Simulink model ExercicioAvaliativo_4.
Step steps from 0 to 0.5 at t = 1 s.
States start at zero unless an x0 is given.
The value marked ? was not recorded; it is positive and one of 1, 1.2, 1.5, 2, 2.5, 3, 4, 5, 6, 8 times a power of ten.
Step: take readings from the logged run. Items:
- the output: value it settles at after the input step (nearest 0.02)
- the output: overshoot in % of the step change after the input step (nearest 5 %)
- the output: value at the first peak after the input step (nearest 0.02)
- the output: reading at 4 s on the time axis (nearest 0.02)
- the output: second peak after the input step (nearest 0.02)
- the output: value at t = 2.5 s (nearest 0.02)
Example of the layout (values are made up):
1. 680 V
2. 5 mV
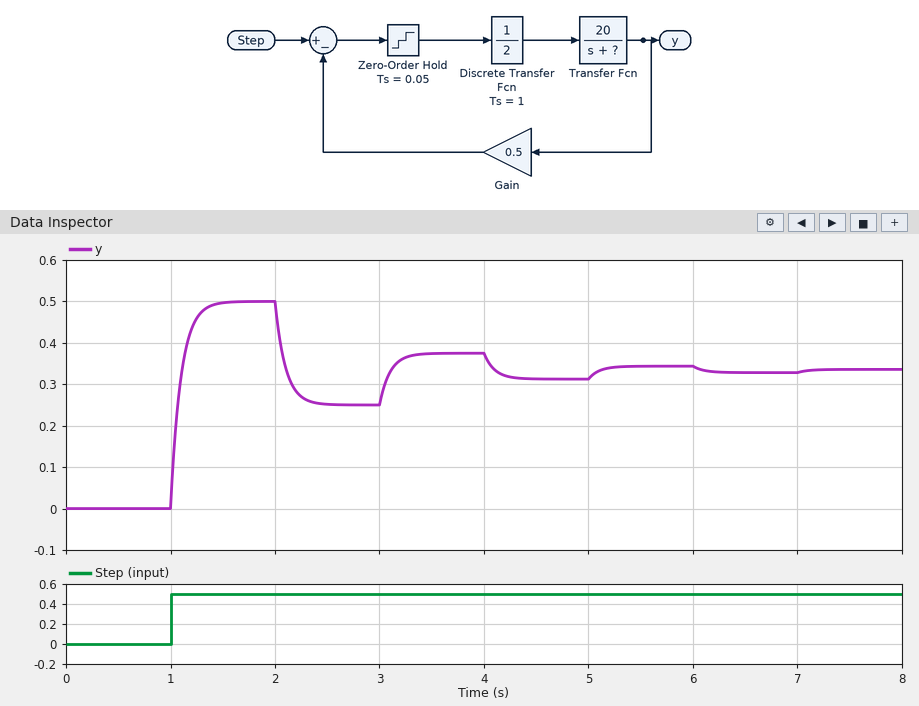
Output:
1. 0.34
2. 50 %
3. 0.50
4. 0.38
5. 0.38
6. 0.26
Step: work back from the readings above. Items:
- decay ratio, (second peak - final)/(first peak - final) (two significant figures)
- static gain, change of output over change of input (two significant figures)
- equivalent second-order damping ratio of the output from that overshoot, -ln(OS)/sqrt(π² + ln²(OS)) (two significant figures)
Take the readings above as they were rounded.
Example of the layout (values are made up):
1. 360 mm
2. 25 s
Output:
1. 0.25
2. 0.68
3. 0.22
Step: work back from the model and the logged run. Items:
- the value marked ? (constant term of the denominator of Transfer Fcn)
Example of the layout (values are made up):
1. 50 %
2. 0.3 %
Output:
1. 10
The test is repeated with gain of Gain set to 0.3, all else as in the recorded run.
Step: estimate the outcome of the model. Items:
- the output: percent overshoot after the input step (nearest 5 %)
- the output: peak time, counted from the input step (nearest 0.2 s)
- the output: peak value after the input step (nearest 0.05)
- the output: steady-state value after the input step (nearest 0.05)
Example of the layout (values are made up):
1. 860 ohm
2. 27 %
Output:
1. 30 %
2. 1.0 s
3. 0.50
4. 0.40
